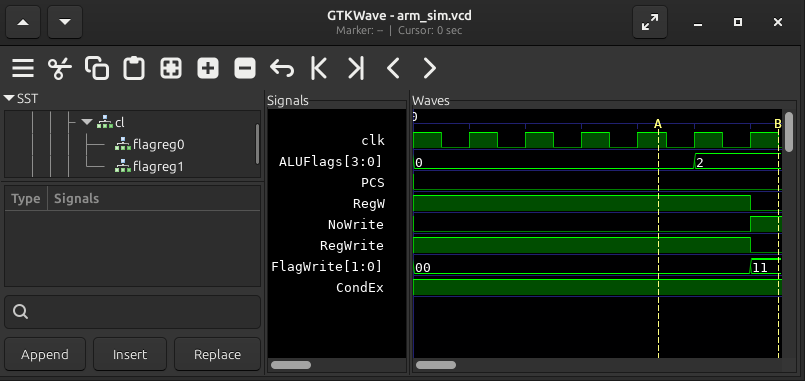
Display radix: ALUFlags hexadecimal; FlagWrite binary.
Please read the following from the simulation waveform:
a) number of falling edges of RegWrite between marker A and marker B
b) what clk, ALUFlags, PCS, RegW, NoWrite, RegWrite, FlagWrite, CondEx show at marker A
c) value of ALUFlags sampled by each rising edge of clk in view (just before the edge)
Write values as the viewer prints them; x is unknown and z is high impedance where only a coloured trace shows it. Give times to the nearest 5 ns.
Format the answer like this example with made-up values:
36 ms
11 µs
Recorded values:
1
clk=1, ALUFlags=0, PCS=0, RegW=1, NoWrite=0, RegWrite=1, FlagWrite=00, CondEx=1
0, 0, 0, 0, 0, 2
